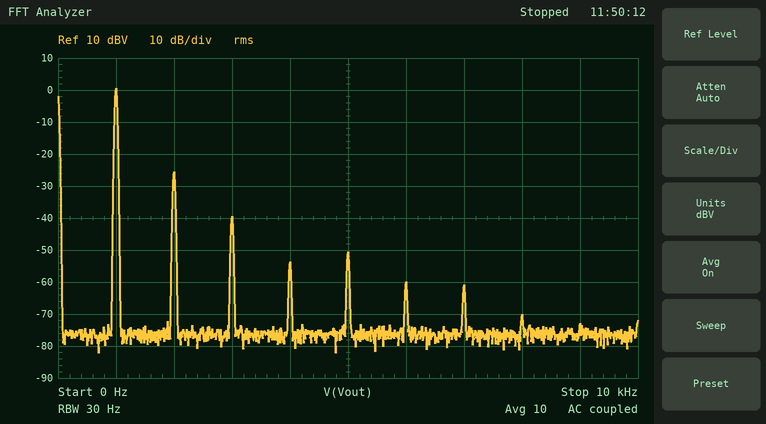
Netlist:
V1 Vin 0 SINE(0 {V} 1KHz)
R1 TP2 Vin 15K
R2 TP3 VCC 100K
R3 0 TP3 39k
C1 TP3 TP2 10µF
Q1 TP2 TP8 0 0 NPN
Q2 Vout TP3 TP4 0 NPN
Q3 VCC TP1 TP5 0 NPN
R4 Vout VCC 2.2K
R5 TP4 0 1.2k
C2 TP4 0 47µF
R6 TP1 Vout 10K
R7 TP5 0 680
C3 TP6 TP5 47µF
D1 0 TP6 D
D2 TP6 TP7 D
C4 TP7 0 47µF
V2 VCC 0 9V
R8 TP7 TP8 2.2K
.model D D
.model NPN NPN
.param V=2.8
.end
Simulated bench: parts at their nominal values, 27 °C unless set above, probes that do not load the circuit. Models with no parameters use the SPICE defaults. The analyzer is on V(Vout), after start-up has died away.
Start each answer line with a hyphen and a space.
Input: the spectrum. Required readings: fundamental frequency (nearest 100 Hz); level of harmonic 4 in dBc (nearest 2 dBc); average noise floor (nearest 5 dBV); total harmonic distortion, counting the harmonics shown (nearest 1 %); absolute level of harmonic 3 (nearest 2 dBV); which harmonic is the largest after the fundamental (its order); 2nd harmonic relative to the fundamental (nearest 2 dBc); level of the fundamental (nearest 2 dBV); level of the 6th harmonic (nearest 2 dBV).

- 1.0 kHz
- -54 dBc
- -75 dBV
- 5 %
- -40 dBV
- 2
- -26 dBc
- 0 dBV
- -60 dBV
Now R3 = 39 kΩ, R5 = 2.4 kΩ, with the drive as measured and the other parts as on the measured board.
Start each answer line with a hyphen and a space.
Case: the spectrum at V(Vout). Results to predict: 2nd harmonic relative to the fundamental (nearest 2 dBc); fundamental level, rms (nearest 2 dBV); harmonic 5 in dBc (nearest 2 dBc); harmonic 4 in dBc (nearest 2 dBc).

- -20 dBc
- 0 dBV
- -52 dBc
- -52 dBc
